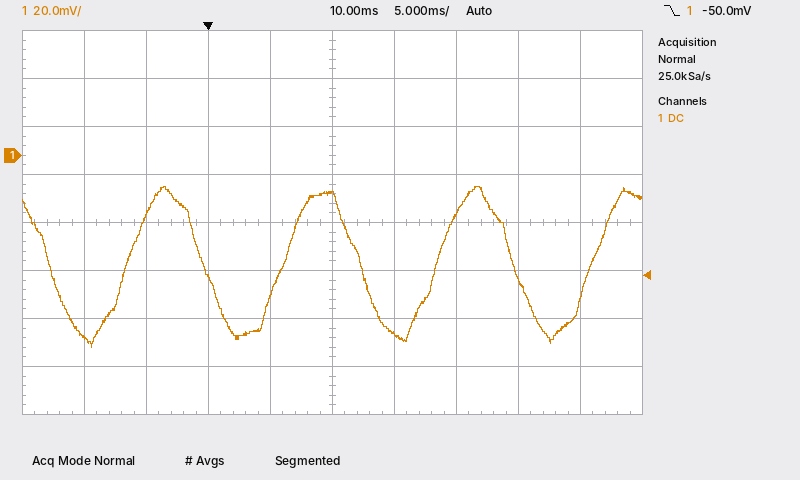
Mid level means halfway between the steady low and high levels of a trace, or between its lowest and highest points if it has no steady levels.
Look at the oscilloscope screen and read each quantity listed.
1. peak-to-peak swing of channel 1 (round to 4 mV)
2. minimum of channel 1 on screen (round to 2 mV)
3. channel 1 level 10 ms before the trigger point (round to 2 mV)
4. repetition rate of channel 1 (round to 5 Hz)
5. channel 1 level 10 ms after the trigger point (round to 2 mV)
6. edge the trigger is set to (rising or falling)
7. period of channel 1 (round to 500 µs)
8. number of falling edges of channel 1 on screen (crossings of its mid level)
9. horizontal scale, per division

68 mV
-80 mV
-76 mV
80 Hz
-16 mV
falling
12.5 ms
4
5 ms
